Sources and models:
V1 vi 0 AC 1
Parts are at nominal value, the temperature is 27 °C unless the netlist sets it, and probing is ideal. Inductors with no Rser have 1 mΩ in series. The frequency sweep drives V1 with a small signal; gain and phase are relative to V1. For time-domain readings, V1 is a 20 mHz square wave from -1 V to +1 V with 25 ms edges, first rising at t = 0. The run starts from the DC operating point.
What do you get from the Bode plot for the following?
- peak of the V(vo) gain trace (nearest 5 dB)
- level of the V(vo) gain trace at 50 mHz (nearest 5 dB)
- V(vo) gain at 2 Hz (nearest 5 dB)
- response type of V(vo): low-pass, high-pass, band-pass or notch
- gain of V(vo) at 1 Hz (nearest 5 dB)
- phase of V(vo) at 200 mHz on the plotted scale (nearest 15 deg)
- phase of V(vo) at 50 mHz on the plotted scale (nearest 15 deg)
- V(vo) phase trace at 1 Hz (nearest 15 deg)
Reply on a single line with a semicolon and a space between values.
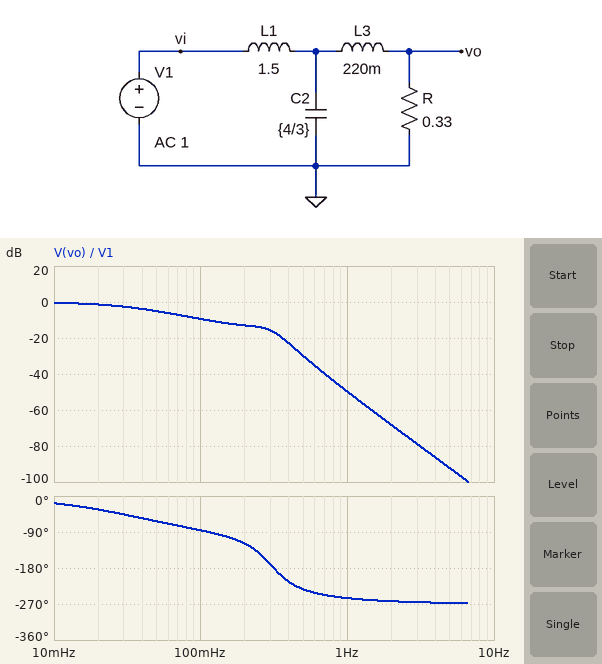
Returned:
0 dB; -5 dB; -70 dB; low-pass; -50 dB; -120 deg; -60 deg; -255 deg
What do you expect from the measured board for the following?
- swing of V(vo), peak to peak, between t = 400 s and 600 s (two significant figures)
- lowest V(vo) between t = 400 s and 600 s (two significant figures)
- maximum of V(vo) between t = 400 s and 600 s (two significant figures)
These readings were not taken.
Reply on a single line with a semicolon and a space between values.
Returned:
2.0 V; -980 mV; 980 mV
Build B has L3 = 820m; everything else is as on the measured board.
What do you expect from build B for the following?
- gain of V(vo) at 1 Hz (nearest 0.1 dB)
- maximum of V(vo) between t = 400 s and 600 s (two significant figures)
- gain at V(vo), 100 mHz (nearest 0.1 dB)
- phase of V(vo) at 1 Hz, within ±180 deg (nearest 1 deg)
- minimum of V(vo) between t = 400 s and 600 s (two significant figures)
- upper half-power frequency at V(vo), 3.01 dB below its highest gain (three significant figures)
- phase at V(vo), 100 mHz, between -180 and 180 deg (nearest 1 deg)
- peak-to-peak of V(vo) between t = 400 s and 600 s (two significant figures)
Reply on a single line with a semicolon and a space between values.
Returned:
-61.5 dB; 950 mV; -10.1 dB; 94 deg; -950 mV; 24.2 mHz; -86 deg; 1.9 V
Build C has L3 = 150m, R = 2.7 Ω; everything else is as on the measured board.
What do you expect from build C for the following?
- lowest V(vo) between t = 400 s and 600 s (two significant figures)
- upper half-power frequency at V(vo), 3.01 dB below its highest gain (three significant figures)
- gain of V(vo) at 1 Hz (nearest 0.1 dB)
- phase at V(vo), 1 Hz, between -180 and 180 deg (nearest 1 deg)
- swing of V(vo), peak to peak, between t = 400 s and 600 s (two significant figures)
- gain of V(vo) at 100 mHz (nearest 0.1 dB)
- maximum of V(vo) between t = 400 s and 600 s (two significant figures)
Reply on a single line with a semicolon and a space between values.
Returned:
-2.1 V; 130 mHz; -38.2 dB; 163 deg; 4.1 V; 7.6 dB; 2.1 V
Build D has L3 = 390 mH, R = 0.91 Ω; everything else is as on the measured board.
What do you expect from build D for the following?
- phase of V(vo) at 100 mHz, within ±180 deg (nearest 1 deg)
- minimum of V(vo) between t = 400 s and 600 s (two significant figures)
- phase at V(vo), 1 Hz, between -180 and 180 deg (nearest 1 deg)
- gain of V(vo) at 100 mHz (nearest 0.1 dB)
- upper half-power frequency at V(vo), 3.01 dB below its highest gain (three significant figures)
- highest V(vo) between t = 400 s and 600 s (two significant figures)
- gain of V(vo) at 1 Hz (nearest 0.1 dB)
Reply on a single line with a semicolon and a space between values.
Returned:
-79 deg; -1.1 V; 111 deg; -0.9 dB; 146 mHz; 1.1 V; -46.6 dB
